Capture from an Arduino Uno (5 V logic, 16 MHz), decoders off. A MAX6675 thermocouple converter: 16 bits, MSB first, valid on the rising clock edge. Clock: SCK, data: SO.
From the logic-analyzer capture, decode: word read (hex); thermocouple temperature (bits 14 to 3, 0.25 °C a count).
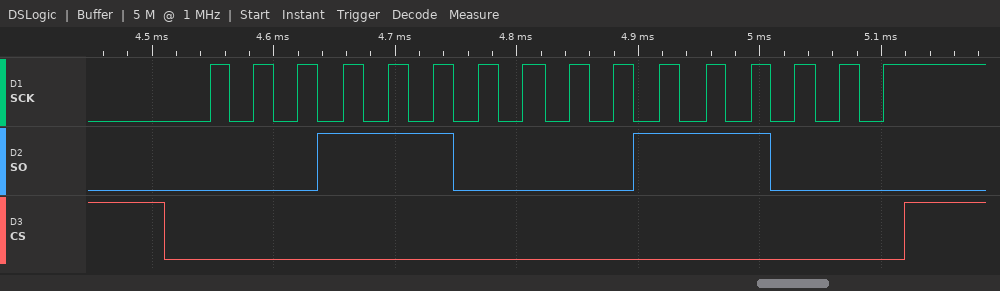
0x1C38
225.75 °C
